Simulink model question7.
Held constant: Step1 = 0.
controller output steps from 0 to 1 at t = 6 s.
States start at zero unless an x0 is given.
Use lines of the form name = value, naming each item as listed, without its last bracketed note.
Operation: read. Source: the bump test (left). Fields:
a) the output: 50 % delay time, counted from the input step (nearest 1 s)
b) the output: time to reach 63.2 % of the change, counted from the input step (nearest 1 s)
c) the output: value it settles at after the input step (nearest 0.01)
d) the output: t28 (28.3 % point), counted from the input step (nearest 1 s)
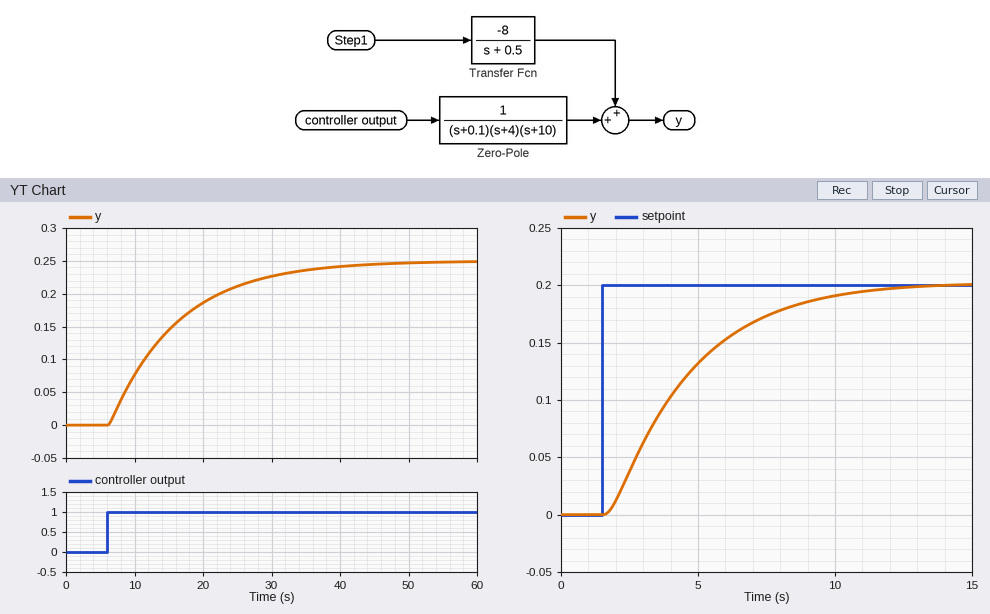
the output: 50 % delay time, counted from the input step = 7 s
the output: time to reach 63.2 % of the change, counted from the input step = 10 s
the output: value it settles at after the input step = 0.25
the output: t28 (28.3 % point), counted from the input step = 4 s
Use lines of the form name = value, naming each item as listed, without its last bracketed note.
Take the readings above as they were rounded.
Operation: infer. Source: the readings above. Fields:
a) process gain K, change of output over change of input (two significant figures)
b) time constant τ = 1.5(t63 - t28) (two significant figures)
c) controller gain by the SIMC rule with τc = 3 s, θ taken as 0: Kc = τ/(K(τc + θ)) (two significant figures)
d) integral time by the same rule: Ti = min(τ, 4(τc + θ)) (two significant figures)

process gain K, change of output over change of input = 0.25
time constant τ = 1.5(t63 - t28) = 9.0 s
controller gain by the SIMC rule with τc = 3 s, θ taken as 0: Kc = τ/(K(τc + θ)) = 12
integral time by the same rule: Ti = min(τ, 4(τc + θ)) = 9.0 s
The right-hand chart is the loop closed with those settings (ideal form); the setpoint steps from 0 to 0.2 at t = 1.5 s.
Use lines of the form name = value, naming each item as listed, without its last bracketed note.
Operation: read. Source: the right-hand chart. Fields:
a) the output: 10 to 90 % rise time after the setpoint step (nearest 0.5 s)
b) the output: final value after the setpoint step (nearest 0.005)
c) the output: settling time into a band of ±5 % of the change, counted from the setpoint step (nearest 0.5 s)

the output: 10 to 90 % rise time after the setpoint step = 6.0 s
the output: final value after the setpoint step = 0.200
the output: settling time into a band of ±5 % of the change, counted from the setpoint step = 8.5 s
